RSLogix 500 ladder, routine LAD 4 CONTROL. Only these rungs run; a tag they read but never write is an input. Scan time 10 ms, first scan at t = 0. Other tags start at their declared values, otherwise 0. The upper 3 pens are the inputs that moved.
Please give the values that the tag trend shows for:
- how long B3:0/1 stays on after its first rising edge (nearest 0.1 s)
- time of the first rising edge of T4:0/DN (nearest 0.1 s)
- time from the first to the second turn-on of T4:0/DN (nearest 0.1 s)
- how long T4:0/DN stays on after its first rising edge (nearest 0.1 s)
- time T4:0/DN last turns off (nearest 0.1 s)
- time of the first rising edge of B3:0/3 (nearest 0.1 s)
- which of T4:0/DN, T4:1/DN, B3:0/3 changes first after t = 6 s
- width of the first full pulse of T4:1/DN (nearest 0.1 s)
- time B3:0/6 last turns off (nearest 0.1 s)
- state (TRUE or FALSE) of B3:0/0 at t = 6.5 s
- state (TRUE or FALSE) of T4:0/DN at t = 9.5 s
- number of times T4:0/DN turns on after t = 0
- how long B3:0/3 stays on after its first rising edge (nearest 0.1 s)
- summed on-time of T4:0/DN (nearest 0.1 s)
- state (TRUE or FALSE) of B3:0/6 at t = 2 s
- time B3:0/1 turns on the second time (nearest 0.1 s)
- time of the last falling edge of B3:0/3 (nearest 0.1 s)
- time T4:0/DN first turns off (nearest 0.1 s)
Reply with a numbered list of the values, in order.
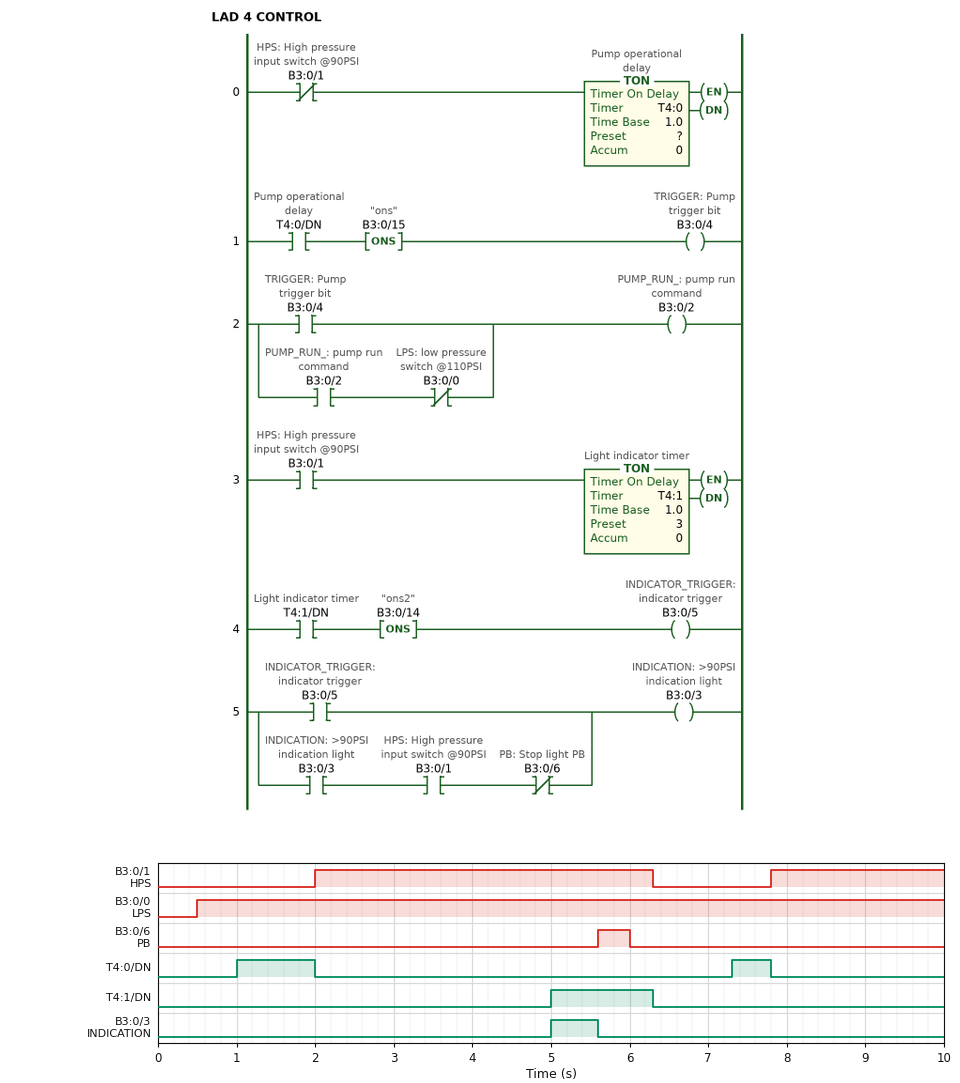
1. 4.3 s
2. 1.0 s
3. 6.3 s
4. 1.0 s
5. 7.8 s
6. 5.0 s
7. T4:1/DN
8. 1.3 s
9. 6.0 s
10. TRUE
11. FALSE
12. 2
13. 0.6 s
14. 1.5 s
15. FALSE
16. 7.8 s
17. 5.6 s
18. 2.0 s
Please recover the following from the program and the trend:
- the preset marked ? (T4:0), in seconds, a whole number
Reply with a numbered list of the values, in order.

1. 1 s
